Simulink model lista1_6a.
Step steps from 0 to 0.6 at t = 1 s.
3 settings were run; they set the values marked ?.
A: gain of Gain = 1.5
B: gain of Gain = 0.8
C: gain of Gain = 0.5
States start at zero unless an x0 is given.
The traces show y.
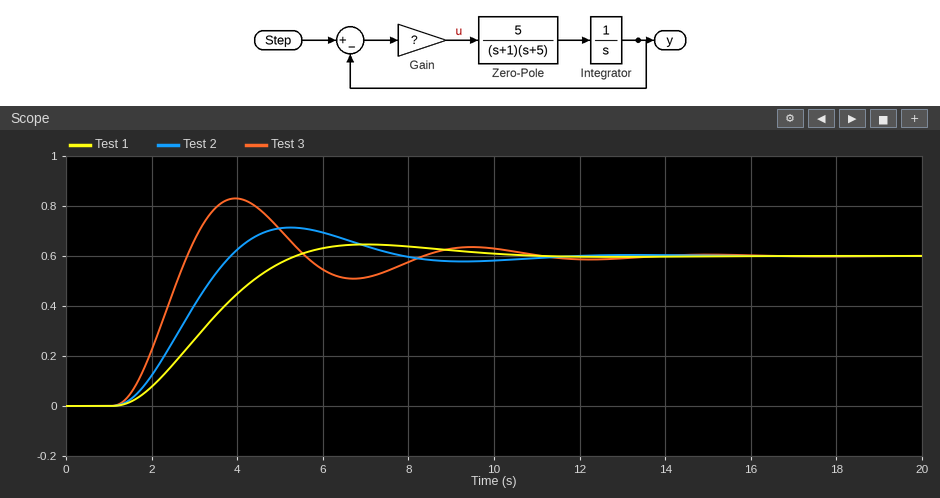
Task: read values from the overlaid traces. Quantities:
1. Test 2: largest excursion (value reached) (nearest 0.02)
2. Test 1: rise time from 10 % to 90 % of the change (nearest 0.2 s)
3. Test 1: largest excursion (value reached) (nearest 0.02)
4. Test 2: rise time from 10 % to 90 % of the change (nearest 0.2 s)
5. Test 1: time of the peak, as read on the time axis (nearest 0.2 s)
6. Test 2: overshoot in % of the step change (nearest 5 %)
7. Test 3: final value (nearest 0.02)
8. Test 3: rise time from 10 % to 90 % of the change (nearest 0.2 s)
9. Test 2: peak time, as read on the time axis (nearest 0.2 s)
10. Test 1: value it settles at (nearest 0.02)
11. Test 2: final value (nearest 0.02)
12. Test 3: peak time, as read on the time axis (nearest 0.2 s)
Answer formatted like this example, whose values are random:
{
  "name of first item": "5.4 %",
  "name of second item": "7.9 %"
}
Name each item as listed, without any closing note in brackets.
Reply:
{
  "Test 2: largest excursion (value reached)": "0.72",
  "Test 1: rise time from 10 % to 90 % of the change": "2.8 s",
  "Test 1: largest excursion (value reached)": "0.64",
  "Test 2: rise time from 10 % to 90 % of the change": "1.8 s",
  "Test 1: time of the peak, as read on the time axis": "7.0 s",
  "Test 2: overshoot in % of the step change": "20 %",
  "Test 3: final value": "0.60",
  "Test 3: rise time from 10 % to 90 % of the change": "1.2 s",
  "Test 2: peak time, as read on the time axis": "5.2 s",
  "Test 1: value it settles at": "0.60",
  "Test 2: final value": "0.60",
  "Test 3: peak time, as read on the time axis": "4.0 s"
}
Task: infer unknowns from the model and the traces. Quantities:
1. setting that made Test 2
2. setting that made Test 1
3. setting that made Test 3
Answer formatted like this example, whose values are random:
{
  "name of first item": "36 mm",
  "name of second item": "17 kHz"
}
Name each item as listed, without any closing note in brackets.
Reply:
{
  "setting that made Test 2": "B",
  "setting that made Test 1": "C",
  "setting that made Test 3": "A"
}
